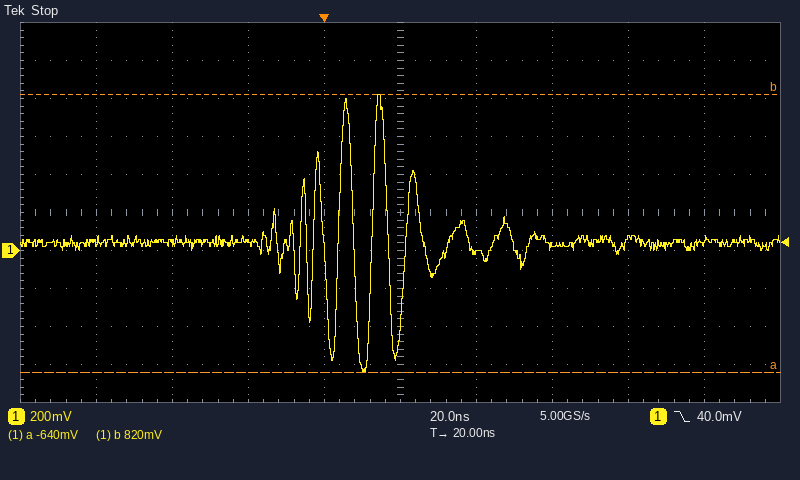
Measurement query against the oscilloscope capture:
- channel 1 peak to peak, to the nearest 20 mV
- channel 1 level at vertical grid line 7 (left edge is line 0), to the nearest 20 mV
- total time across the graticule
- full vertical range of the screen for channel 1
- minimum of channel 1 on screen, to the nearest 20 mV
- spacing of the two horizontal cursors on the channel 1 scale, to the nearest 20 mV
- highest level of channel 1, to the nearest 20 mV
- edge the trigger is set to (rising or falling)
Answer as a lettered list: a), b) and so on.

a) 1.46 V
b) 20 mV
c) 200 ns
d) 2 V
e) -640 mV
f) 1.46 V
g) 820 mV
h) falling
